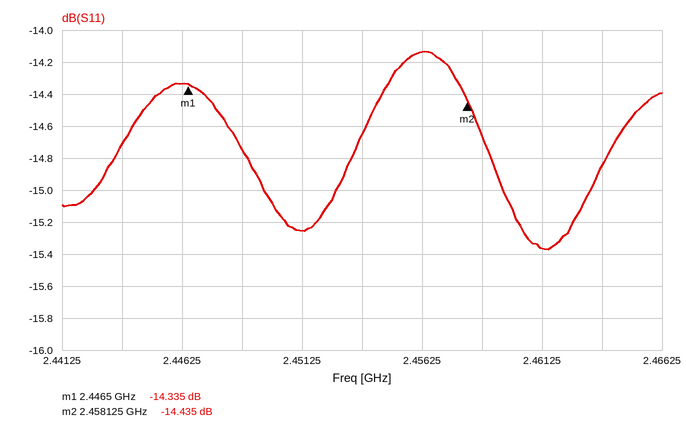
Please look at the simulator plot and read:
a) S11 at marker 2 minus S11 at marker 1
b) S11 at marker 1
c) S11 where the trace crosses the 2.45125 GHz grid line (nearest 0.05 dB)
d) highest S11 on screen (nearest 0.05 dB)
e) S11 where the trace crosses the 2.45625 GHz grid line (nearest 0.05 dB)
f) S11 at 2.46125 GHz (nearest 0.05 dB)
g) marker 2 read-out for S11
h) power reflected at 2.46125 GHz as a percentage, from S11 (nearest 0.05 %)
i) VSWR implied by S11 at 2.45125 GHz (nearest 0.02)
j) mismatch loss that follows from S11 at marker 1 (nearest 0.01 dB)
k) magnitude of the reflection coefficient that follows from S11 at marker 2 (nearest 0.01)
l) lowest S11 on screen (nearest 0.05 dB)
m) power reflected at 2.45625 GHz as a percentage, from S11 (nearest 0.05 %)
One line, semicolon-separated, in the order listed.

-0.100 dB; -14.335 dB; -15.25 dB; -14.15 dB; -14.15 dB; -15.35 dB; -14.435 dB; 2.90 %; 1.42; 0.16 dB; 0.19; -15.35 dB; 3.85 %
